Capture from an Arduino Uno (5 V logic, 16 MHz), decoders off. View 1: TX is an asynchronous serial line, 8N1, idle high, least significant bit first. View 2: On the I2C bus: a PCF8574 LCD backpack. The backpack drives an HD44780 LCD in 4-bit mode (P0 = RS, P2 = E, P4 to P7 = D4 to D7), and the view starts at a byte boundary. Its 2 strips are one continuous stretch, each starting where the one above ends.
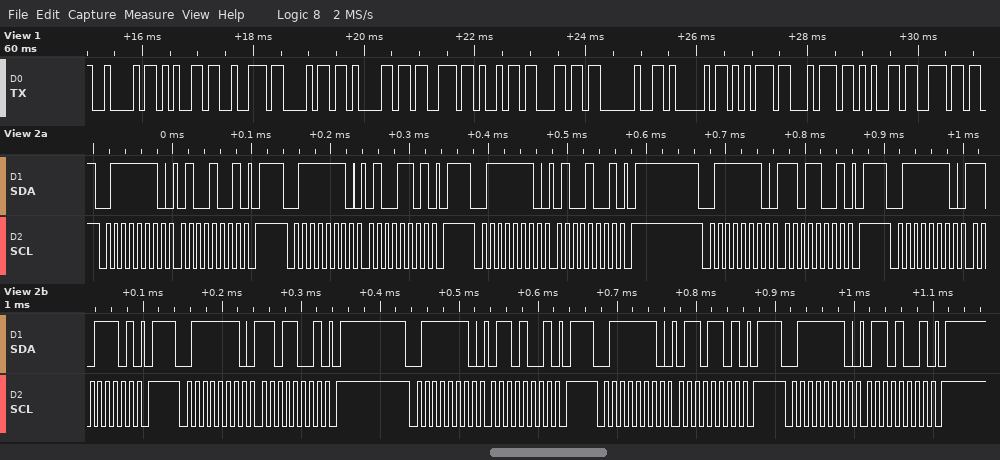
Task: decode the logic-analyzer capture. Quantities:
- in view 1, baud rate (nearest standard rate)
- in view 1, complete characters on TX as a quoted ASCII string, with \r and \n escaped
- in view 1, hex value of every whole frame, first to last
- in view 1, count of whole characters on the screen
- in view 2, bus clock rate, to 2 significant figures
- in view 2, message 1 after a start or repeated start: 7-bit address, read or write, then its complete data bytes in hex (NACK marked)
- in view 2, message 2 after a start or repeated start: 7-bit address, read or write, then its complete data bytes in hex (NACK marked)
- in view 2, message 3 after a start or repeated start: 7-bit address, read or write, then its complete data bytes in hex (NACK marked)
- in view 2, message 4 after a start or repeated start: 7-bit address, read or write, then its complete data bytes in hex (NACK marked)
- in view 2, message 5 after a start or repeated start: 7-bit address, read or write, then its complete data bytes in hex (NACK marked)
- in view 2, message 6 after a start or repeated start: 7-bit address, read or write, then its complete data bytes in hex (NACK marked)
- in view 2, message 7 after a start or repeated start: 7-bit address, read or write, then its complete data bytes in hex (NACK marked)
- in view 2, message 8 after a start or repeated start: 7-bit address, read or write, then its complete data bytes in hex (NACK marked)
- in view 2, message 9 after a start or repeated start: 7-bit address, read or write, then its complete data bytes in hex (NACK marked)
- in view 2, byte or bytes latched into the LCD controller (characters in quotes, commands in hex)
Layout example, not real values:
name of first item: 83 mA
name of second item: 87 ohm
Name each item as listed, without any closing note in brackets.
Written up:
in view 1, baud rate: 9600 baud
in view 1, complete characters on TX as a quoted ASCII string, with \r and \n escaped: "Berhasil Auten"
in view 1, hex value of every whole frame, first to last: 42 65 72 68 61 73 69 6C 20 41 75 74 65 6E
in view 1, count of whole characters on the screen: 14
in view 2, bus clock rate, to 2 significant figures: 100 kHz
in view 2, message 1 after a start or repeated start: 7-bit address, read or write, then its complete data bytes in hex: 0x3F write: 49
in view 2, message 2 after a start or repeated start: 7-bit address, read or write, then its complete data bytes in hex: 0x3F write: 4D
in view 2, message 3 after a start or repeated start: 7-bit address, read or write, then its complete data bytes in hex: 0x3F write: 49
in view 2, message 4 after a start or repeated start: 7-bit address, read or write, then its complete data bytes in hex: 0x3F write: D9
in view 2, message 5 after a start or repeated start: 7-bit address, read or write, then its complete data bytes in hex: 0x3F write: DD
in view 2, message 6 after a start or repeated start: 7-bit address, read or write, then its complete data bytes in hex: 0x3F write: D9
in view 2, message 7 after a start or repeated start: 7-bit address, read or write, then its complete data bytes in hex: 0x3F write: 69
in view 2, message 8 after a start or repeated start: 7-bit address, read or write, then its complete data bytes in hex: 0x3F write: 6D
in view 2, message 9 after a start or repeated start: 7-bit address, read or write, then its complete data bytes in hex: 0x3F write: 69
in view 2, byte or bytes latched into the LCD controller: 'M'
